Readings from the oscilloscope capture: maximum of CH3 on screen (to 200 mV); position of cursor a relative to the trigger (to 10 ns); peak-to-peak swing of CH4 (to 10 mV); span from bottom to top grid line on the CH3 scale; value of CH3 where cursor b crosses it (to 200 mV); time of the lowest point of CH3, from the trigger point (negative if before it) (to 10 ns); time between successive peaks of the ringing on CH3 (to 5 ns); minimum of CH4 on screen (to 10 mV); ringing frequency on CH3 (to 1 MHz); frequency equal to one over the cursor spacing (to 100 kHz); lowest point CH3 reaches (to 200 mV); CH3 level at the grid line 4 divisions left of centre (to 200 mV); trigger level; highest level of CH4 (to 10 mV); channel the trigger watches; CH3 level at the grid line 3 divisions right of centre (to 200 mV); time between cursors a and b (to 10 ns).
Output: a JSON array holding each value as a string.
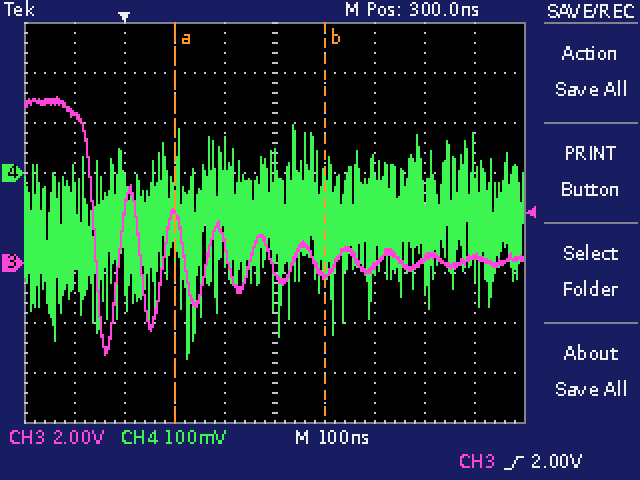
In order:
["6.6 V", "+100 ns", "470 mV", "16 V", "-400 mV", "-40 ns", "85 ns", "-370 mV", "12 MHz", "3.3 MHz", "-3.6 V", "6.0 V", "2.00 V", "100 mV", "CH3", "200 mV", "300 ns"]
